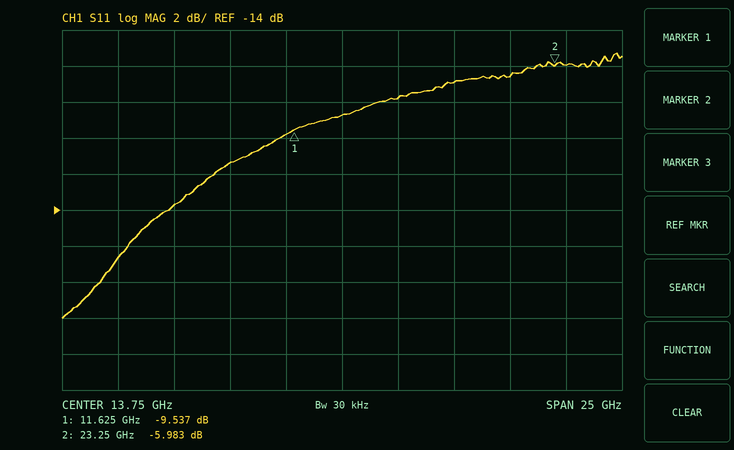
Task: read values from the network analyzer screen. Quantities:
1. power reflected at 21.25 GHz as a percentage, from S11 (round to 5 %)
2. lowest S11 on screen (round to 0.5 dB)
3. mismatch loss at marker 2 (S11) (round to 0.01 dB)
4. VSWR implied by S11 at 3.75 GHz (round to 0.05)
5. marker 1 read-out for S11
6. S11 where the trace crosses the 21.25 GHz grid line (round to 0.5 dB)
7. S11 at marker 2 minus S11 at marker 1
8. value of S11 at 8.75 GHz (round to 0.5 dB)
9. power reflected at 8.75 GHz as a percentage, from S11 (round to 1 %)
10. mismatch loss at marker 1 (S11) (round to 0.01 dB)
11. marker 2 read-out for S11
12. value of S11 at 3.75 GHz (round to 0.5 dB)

20 %
-20.0 dB
1.26 dB
1.35
-9.537 dB
-6.5 dB
3.554 dB
-11.5 dB
7 %
0.51 dB
-5.983 dB
-16.5 dB
